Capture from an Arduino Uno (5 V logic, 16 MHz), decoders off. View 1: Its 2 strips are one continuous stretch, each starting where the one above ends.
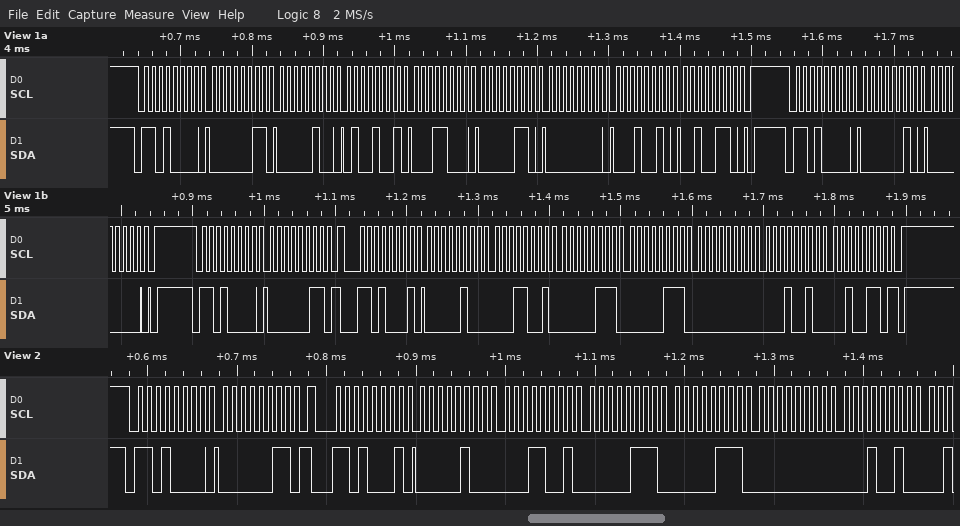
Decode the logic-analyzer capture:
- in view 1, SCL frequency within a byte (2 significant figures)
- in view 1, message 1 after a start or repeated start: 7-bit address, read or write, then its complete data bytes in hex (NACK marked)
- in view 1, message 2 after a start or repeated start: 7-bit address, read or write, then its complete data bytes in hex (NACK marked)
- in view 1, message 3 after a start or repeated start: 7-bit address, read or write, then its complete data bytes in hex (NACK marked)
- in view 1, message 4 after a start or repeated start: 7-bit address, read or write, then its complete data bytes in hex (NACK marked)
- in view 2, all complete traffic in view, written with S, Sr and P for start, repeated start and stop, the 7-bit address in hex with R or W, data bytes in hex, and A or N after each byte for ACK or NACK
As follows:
100 kHz
0x68 write: 03 04 49 18 06 00 12 26
0x68 write: 02 00
0x68 write: 03
0x68 read: 04 19 07 07 00 12 26 NACK
S 68W A 03 A Sr 68R A 04 A 19 A 07 A 07 A 00 A 12 A
